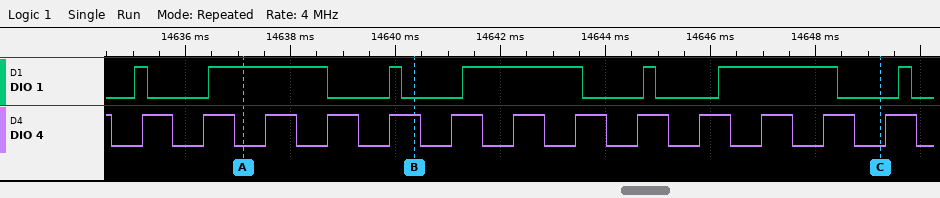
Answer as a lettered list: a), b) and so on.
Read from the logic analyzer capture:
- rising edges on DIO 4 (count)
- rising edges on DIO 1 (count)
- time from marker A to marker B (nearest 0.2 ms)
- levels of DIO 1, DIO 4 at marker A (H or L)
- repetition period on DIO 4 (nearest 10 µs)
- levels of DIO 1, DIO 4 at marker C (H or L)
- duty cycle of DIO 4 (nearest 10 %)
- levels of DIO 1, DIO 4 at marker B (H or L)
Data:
a) 13
b) 7
c) 3.2 ms
d) DIO 1=H, DIO 4=L
e) 1180 µs
f) DIO 1=L, DIO 4=L
g) 50 %
h) DIO 1=L, DIO 4=H
